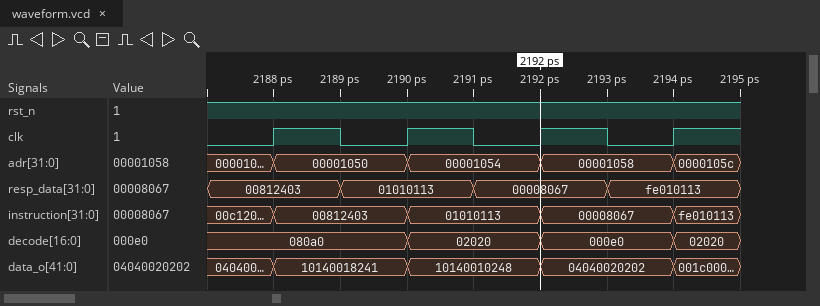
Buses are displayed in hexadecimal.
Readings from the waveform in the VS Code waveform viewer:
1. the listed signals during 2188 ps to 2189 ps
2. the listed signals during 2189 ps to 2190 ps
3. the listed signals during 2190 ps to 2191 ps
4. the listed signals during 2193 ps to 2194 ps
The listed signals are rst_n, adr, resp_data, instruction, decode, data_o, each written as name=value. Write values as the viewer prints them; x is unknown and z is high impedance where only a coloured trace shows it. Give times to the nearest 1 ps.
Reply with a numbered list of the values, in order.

1. rst_n=1, adr=00001050, resp_data=00812403, instruction=00812403, decode=080a0, data_o=10140018241
2. rst_n=1, adr=00001050, resp_data=01010113, instruction=00812403, decode=080a0, data_o=10140018241
3. rst_n=1, adr=00001054, resp_data=01010113, instruction=01010113, decode=02020, data_o=10140010248
4. rst_n=1, adr=00001058, resp_data=fe010113, instruction=00008067, decode=000e0, data_o=04040020202
